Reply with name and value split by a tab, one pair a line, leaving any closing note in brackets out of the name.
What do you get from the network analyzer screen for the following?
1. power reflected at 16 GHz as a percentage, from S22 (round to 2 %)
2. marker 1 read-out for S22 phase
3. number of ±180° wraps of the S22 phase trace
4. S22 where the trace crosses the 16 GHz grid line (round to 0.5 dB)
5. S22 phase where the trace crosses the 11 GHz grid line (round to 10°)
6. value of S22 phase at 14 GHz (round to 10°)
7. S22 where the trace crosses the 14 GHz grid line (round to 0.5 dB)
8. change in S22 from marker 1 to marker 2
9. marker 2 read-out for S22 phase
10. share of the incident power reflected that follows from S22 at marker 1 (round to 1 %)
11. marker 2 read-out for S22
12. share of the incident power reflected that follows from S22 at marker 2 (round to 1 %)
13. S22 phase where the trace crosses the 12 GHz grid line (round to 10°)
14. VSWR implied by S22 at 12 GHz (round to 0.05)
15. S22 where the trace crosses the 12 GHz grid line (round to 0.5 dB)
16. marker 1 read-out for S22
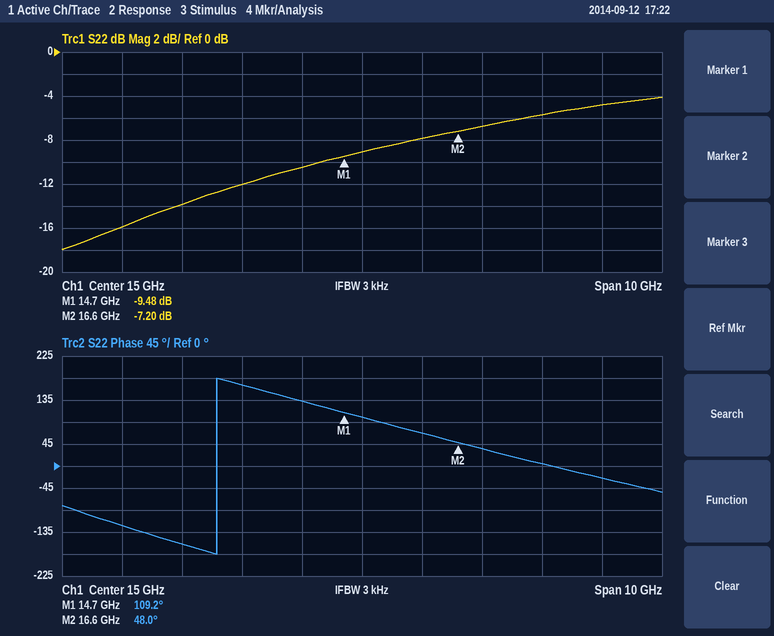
power reflected at 16 GHz as a percentage, from S22	16 %
marker 1 read-out for S22 phase	109.2°
number of ±180° wraps of the S22 phase trace	1
S22 where the trace crosses the 16 GHz grid line	-8.0 dB
S22 phase where the trace crosses the 11 GHz grid line	-120°
value of S22 phase at 14 GHz	130°
S22 where the trace crosses the 14 GHz grid line	-10.5 dB
change in S22 from marker 1 to marker 2	2.28 dB
marker 2 read-out for S22 phase	48.0°
share of the incident power reflected that follows from S22 at marker 1	11 %
marker 2 read-out for S22	-7.20 dB
share of the incident power reflected that follows from S22 at marker 2	19 %
S22 phase where the trace crosses the 12 GHz grid line	-160°
VSWR implied by S22 at 12 GHz	1.50
S22 where the trace crosses the 12 GHz grid line	-14.0 dB
marker 1 read-out for S22	-9.48 dB
